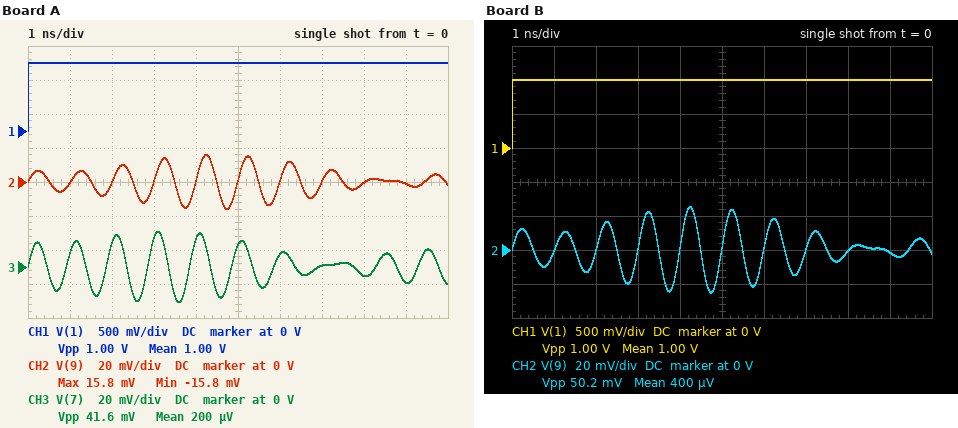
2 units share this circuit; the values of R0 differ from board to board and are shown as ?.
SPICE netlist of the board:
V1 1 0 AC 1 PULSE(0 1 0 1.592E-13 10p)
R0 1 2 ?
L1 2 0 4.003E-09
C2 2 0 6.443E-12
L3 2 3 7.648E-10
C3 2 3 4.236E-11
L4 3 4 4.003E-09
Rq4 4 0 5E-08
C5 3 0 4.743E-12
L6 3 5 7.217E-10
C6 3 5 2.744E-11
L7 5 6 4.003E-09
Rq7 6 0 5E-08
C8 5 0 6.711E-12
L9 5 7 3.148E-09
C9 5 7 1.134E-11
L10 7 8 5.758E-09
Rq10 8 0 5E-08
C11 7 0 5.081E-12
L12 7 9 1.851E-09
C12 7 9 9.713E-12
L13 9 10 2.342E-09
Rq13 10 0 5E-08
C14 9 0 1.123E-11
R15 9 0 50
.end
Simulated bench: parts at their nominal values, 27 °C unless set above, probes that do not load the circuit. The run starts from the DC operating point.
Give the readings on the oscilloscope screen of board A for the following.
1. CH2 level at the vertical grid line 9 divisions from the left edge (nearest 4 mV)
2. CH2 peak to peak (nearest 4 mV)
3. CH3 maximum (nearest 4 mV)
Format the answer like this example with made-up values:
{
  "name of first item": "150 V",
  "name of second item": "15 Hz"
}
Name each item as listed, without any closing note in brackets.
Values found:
{
  "CH2 level at the vertical grid line 9 divisions from the left edge": "0 V",
  "CH2 peak to peak": "32 mV",
  "CH3 maximum": "20 mV"
}
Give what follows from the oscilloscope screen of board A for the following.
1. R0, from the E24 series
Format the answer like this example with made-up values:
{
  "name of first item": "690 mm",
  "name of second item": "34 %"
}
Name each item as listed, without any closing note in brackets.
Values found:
{
  "R0, from the E24 series": "160 Ω"
}
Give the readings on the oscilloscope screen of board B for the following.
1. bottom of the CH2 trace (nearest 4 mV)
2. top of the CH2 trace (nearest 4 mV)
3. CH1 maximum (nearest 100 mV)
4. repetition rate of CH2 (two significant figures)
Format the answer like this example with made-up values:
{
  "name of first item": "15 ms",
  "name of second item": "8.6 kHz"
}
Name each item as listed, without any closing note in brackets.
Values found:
{
  "bottom of the CH2 trace": "-24 mV",
  "top of the CH2 trace": "24 mV",
  "CH1 maximum": "1.0 V",
  "repetition rate of CH2": "1.0 GHz"
}
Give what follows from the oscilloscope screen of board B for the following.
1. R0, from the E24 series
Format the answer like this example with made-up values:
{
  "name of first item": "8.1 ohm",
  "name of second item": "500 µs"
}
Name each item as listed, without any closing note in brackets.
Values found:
{
  "R0, from the E24 series": "82 Ω"
}
